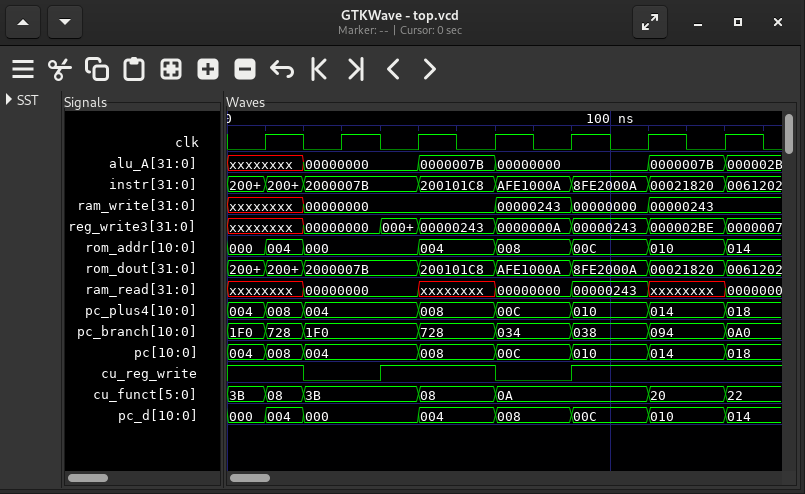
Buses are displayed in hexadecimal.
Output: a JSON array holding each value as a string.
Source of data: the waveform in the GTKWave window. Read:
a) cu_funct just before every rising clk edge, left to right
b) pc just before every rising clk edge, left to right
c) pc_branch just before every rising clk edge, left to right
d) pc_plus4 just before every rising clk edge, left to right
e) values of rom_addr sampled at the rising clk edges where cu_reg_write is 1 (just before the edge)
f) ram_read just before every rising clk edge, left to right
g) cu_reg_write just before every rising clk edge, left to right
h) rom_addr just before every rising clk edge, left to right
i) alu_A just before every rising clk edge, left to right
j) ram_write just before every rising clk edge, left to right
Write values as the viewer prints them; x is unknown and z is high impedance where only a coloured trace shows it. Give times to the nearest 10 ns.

["3B, 3B, 3B, 08, 0A, 0A, 20", "004, 004, 004, 008, 00C, 010, 014", "1F0, 1F0, 1F0, 728, 034, 038, 094", "004, 004, 004, 008, 00C, 010, 014", "000, 000, 004, 00C, 010", "xxxxxxxx, 00000000, 00000000, xxxxxxxx, 00000000, 00000243, xxxxxxxx", "1 0 1 1 0 1 1", "000, 000, 000, 004, 008, 00C, 010", "xxxxxxxx, 00000000, 00000000, 0000007B, 00000000, 00000000, 0000007B", "xxxxxxxx, 00000000, 00000000, 00000000, 00000243, 00000000, 00000243"]
